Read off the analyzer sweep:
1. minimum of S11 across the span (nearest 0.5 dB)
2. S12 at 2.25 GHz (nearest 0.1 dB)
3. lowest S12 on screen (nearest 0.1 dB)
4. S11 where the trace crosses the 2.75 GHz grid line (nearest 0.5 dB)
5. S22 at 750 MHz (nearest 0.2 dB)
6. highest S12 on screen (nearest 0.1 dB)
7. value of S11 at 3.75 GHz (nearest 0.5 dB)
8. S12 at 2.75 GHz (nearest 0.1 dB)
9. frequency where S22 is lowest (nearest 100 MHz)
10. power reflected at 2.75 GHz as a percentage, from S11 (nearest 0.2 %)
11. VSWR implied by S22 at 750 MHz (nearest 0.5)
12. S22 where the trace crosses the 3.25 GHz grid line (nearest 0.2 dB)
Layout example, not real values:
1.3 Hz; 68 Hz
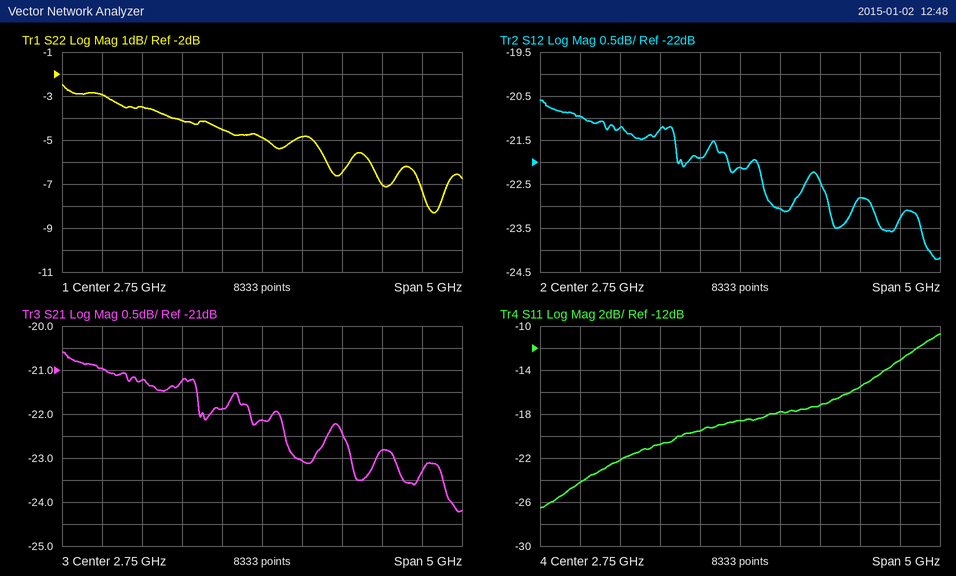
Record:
-26.5 dB; -21.9 dB; -24.2 dB; -18.5 dB; -3.0 dB; -20.6 dB; -17.0 dB; -22.1 dB; 4.9 GHz; 1.4 %; 6.0; -4.8 dB
